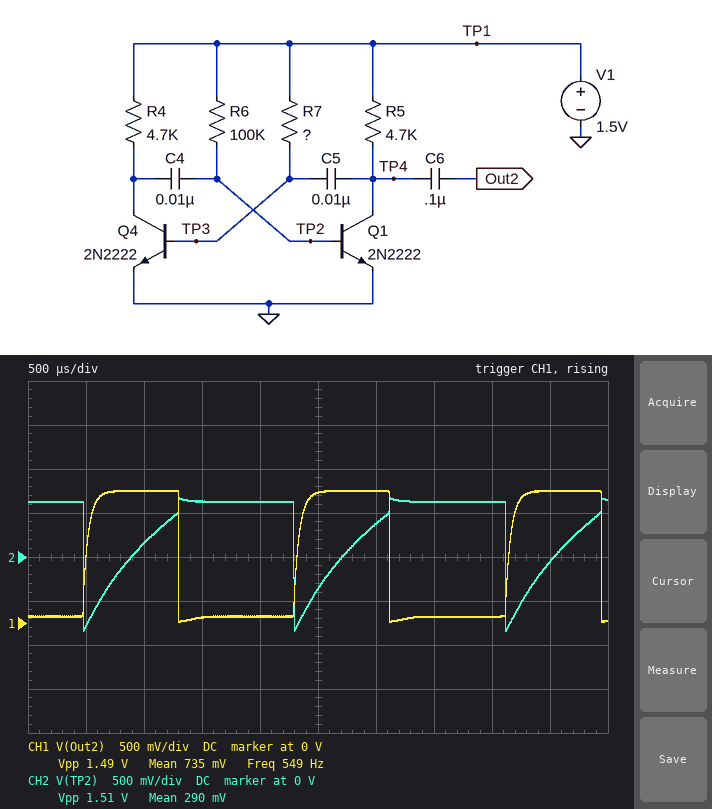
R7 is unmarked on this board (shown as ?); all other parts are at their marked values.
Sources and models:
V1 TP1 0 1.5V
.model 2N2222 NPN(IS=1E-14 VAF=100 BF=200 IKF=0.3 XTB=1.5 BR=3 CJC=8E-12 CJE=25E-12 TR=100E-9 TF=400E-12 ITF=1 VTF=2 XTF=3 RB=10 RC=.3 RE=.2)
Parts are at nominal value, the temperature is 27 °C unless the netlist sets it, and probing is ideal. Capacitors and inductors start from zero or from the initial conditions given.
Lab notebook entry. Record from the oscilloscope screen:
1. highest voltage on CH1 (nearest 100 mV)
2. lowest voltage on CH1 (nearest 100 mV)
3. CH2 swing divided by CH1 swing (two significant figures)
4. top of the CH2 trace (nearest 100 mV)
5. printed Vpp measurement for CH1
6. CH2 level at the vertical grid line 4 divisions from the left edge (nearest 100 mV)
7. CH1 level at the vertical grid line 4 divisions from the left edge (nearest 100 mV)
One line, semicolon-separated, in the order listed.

1.5 V; 0 V; 1.0; 700 mV; 1.49 V; 600 mV; 100 mV
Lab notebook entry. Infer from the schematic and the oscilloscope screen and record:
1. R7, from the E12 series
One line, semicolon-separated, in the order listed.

120 kΩ
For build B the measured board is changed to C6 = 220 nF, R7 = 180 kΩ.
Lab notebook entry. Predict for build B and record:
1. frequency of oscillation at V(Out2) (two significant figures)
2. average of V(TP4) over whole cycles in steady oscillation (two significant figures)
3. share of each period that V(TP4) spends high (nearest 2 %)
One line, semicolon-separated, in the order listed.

430 Hz; 540 mV; 34 %
